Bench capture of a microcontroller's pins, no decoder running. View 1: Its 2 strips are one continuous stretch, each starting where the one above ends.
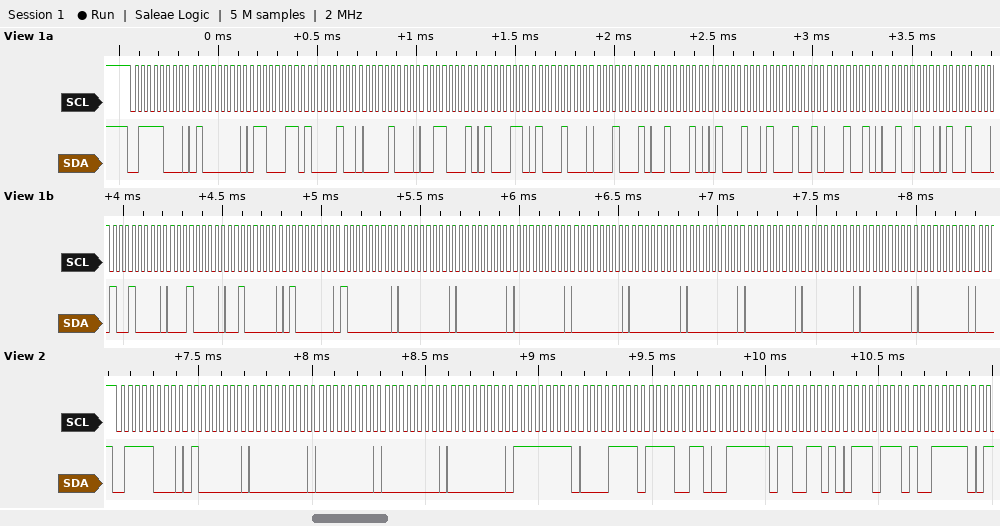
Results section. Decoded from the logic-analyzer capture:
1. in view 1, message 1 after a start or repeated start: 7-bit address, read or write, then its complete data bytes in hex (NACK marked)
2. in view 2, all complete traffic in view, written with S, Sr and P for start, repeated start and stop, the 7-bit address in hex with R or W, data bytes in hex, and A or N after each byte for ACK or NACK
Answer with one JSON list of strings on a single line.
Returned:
["0x3C write: 40 63 84 08 31 46 88 11 22 44 89 12 24 48 90 10 20 40 80 00 00 00 00 00 00 00 00 00 00", "S 3CW A 40 A 00 A 00 A 00 A 00 A FF A 0F A F3 A 3F A CD A 77 A 9F A"]
